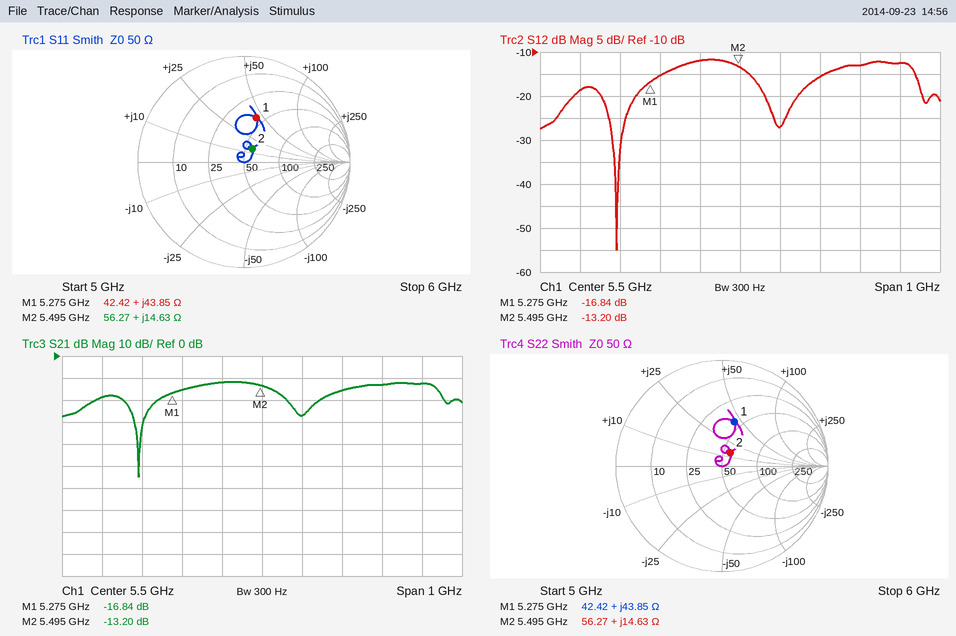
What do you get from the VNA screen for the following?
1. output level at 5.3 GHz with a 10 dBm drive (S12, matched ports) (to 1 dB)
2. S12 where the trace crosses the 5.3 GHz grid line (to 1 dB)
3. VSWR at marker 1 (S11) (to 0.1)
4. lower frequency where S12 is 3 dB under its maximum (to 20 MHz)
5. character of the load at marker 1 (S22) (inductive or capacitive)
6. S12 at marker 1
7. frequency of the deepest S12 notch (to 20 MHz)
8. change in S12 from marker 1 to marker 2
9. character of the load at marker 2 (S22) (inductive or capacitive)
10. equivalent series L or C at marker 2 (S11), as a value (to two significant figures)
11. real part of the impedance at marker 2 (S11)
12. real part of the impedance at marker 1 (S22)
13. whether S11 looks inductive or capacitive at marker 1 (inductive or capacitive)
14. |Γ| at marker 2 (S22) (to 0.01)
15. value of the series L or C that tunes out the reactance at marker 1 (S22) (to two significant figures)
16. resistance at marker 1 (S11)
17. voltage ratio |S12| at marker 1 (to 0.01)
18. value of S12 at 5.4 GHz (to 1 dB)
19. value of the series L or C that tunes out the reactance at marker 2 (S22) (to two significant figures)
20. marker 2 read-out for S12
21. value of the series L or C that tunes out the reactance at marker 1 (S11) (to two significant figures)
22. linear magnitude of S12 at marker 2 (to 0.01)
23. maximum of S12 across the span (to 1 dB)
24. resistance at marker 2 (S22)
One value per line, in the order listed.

-5 dBm
-15 dB
2.5
5.32 GHz
inductive
-16.84 dB
5.20 GHz
3.64 dB
inductive
420 pH
56.27 Ω
42.42 Ω
inductive
0.15
690 fF
42.42 Ω
0.14
-12 dB
2.0 pF
-13.20 dB
690 fF
0.22
-12 dB
56.27 Ω
